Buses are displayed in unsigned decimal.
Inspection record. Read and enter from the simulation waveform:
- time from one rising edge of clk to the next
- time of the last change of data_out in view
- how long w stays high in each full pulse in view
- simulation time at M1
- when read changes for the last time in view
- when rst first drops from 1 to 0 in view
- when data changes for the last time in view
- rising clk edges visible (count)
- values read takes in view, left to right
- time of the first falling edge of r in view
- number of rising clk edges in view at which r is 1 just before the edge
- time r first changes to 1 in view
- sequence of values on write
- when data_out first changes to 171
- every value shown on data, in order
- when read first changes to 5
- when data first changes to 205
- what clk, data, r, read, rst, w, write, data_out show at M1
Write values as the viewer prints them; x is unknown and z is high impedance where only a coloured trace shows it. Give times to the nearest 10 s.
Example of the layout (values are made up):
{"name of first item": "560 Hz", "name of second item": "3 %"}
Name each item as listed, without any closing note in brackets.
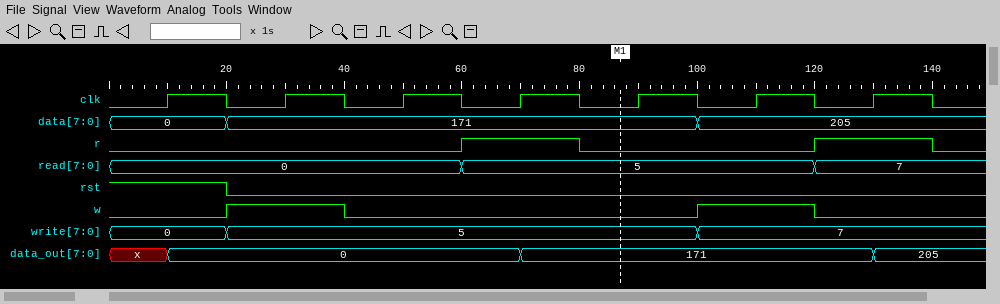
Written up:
{"time from one rising edge of clk to the next": "20 s", "time of the last change of data_out in view": "130 s", "how long w stays high in each full pulse in view": "20 s, 20 s", "simulation time at M1": "90 s", "when read changes for the last time in view": "120 s", "when rst first drops from 1 to 0 in view": "20 s", "when data changes for the last time in view": "100 s", "rising clk edges visible": "7", "values read takes in view, left to right": "0, 5, 7", "time of the first falling edge of r in view": "80 s", "number of rising clk edges in view at which r is 1 just before the edge": "2", "time r first changes to 1 in view": "60 s", "sequence of values on write": "0, 5, 7", "when data_out first changes to 171": "70 s", "every value shown on data, in order": "0, 171, 205", "when read first changes to 5": "60 s", "when data first changes to 205": "100 s", "what clk, data, r, read, rst, w, write, data_out show at M1": "clk=0, data=171, r=0, read=5, rst=0, w=0, write=5, data_out=171"}
